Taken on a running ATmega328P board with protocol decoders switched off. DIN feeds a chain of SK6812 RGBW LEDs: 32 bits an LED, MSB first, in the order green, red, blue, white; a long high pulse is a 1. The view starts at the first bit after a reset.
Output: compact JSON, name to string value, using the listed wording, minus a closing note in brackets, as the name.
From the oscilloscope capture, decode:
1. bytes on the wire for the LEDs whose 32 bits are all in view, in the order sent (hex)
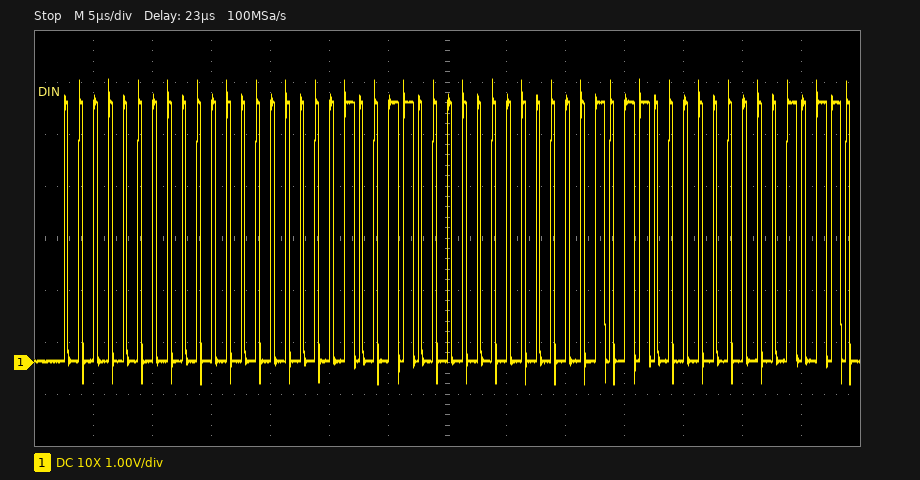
{"bytes on the wire for the LEDs whose 32 bits are all in view, in the order sent": "00 00 13 00"}
